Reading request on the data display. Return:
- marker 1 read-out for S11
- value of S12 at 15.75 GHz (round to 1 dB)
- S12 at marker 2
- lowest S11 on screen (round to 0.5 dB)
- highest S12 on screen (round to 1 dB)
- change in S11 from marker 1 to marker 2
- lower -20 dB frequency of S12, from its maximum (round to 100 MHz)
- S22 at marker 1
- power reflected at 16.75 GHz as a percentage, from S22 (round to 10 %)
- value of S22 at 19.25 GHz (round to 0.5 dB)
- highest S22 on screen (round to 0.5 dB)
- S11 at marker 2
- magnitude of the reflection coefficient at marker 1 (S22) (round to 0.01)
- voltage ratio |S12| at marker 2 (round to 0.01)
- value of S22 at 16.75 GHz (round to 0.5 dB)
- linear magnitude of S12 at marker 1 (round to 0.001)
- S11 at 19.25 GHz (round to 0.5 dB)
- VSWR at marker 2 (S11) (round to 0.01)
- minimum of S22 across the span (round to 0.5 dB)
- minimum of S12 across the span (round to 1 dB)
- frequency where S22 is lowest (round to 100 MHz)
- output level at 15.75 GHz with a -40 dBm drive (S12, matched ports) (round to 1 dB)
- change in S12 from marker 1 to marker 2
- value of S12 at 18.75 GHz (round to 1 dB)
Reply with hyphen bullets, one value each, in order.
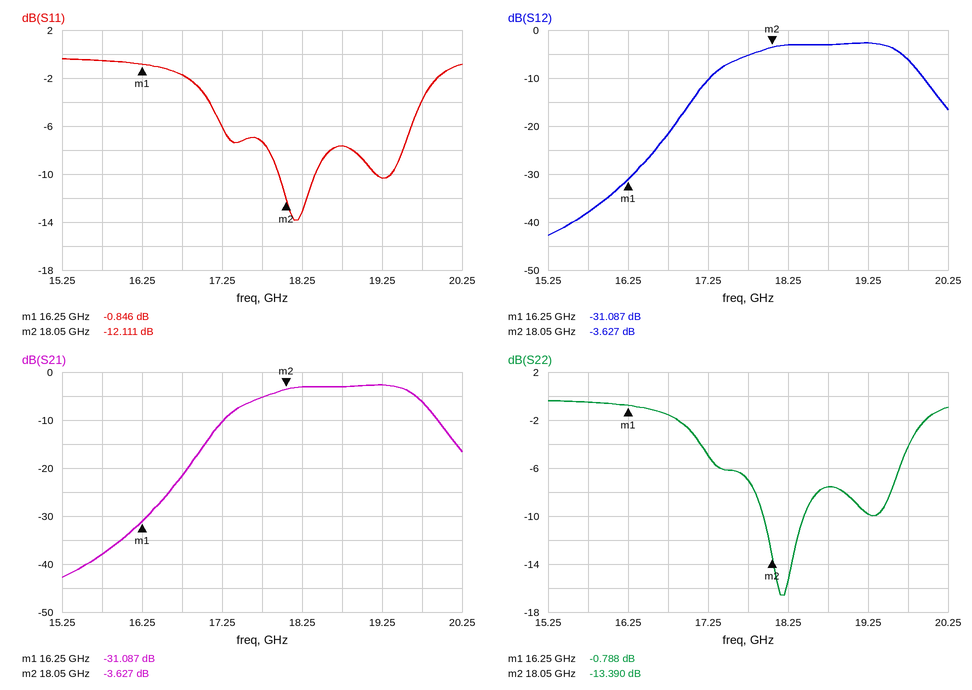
- -0.846 dB
- -38 dB
- -3.627 dB
- -14.0 dB
- -3 dB
- -11.265 dB
- 16.7 GHz
- -0.788 dB
- 70 %
- -10.0 dB
- -0.5 dB
- -12.111 dB
- 0.91
- 0.66
- -1.5 dB
- 0.028
- -10.5 dB
- 1.66
- -16.5 dB
- -43 dB
- 18.2 GHz
- -78 dBm
- 27.460 dB
- -3 dB
